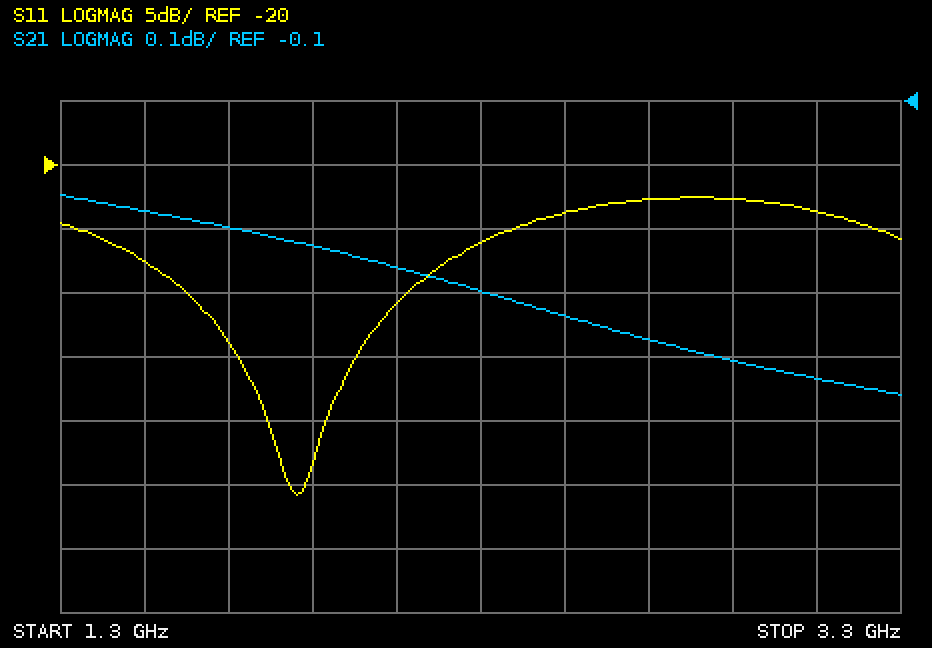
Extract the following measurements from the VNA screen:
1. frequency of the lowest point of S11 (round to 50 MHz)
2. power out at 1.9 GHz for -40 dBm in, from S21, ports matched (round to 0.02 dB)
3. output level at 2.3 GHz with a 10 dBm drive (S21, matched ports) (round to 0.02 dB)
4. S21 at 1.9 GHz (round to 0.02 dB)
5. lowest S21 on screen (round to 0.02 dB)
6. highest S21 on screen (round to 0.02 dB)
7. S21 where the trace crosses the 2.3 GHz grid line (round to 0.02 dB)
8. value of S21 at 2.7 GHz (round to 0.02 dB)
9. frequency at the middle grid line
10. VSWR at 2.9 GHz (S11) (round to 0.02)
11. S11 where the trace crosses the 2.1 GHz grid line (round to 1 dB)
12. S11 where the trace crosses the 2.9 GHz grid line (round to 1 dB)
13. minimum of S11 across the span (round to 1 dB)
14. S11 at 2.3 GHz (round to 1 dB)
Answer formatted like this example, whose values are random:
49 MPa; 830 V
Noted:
1.85 GHz; -40.32 dBm; 9.60 dBm; -0.32 dB; -0.56 dB; -0.24 dB; -0.40 dB; -0.48 dB; 2.3 GHz; 1.16; -31 dB; -23 dB; -46 dB; -26 dB
